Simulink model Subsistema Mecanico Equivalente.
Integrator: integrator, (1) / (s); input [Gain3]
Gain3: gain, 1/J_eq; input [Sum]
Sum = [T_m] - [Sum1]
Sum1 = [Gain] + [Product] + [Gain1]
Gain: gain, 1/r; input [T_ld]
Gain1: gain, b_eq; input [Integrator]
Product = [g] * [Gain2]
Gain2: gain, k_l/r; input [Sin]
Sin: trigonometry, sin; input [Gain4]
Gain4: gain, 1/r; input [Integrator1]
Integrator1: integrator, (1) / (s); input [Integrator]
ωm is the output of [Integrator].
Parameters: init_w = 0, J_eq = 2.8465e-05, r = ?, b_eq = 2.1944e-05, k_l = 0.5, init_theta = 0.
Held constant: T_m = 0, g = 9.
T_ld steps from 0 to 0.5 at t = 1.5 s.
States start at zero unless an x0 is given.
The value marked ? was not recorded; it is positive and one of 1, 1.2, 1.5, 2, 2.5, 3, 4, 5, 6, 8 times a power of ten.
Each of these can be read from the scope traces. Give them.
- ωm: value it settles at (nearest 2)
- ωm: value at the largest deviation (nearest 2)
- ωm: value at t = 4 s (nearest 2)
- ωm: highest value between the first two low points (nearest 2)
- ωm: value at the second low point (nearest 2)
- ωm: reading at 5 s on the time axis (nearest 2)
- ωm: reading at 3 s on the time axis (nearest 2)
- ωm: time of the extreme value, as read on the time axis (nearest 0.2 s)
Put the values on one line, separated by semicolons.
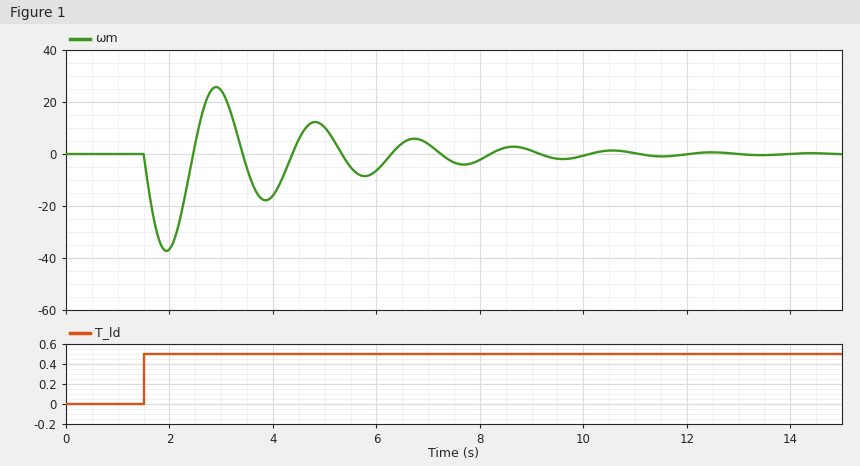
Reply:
0; -38; -16; 26; -18; 10; 24; 2.0 s
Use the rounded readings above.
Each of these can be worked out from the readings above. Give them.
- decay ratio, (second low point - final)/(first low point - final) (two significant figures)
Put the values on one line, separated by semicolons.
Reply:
0.47
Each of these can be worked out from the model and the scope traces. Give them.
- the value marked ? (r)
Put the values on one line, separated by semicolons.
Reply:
120
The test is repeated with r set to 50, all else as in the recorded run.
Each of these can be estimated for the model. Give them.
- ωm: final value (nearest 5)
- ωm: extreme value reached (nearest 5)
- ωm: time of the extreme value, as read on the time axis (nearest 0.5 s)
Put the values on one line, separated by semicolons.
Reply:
0; -40; 1.5 s
